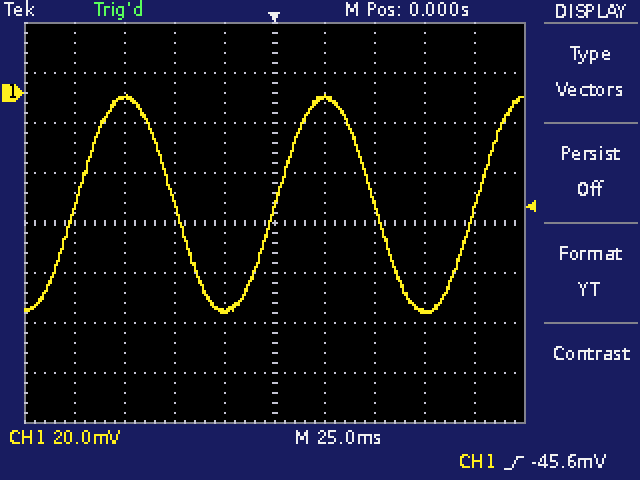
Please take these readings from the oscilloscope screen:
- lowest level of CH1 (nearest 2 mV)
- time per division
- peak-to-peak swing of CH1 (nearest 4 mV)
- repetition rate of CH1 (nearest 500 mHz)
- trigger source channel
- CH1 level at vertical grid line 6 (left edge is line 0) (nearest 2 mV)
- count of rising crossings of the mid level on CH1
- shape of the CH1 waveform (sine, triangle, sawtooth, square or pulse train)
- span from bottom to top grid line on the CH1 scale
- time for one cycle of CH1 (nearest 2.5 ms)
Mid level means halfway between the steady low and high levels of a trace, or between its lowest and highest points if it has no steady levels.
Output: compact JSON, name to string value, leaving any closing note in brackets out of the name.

{"lowest level of CH1": "-88 mV", "time per division": "25 ms", "peak-to-peak swing of CH1": "88 mV", "repetition rate of CH1": "10.0 Hz", "trigger source channel": "CH1", "CH1 level at vertical grid line 6 (left edge is line 0)": "-2 mV", "count of rising crossings of the mid level on CH1": "3", "shape of the CH1 waveform": "sine", "span from bottom to top grid line on the CH1 scale": "160 mV", "time for one cycle of CH1": "100.0 ms"}
